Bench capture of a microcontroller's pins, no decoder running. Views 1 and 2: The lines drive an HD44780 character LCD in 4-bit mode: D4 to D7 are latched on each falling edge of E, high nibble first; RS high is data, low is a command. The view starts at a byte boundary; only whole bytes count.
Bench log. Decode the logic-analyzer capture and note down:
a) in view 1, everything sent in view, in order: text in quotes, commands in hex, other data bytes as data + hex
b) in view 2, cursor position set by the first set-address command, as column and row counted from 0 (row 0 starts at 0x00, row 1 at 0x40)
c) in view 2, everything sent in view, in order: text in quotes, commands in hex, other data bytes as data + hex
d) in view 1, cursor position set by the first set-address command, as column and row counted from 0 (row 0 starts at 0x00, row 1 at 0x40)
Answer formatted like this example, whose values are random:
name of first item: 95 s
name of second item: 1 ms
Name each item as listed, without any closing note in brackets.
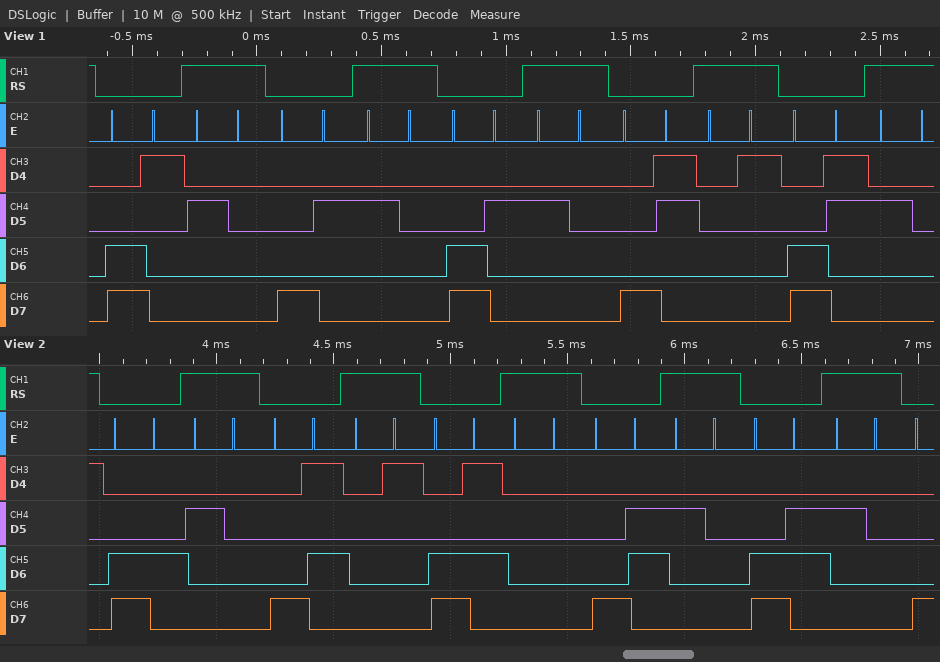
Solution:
in view 1, everything sent in view, in order: text in quotes, commands in hex, other data bytes as data + hex: 0xC1 " " 0x82 " " 0xC2 " " 0x83 data 01 0xC3 " "
in view 2, cursor position set by the first set-address command, as column and row counted from 0: column 4, row 1
in view 2, everything sent in view, in order: text in quotes, commands in hex, other data bytes as data + hex: 0xC4 " " 0x85 data 01 0xC5 data 00 0x86 " " 0xC6 " "
in view 1, cursor position set by the first set-address command, as column and row counted from 0: column 1, row 1
